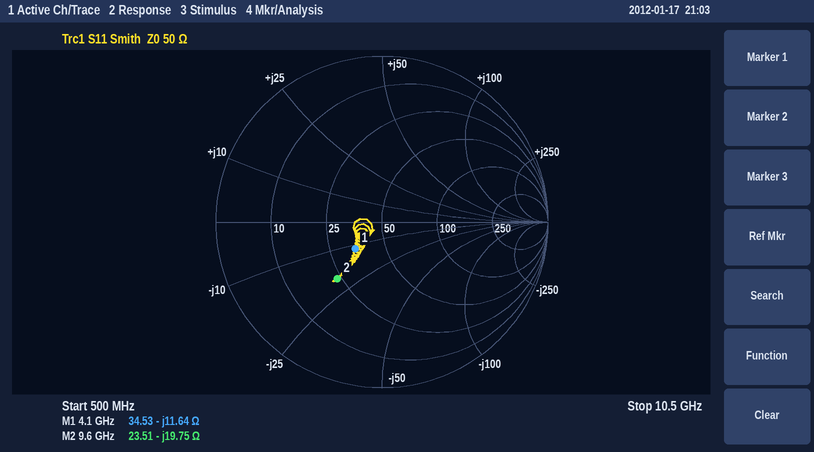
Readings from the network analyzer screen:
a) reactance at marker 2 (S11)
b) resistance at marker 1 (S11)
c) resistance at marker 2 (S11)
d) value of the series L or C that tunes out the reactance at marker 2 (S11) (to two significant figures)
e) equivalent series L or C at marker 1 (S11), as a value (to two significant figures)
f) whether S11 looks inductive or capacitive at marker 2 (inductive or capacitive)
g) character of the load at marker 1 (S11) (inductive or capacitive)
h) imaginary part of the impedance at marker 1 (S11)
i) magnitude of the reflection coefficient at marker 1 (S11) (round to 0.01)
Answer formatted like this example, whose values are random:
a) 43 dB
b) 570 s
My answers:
a) -19.75 Ω
b) 34.53 Ω
c) 23.51 Ω
d) 330 pH
e) 3.3 pF
f) capacitive
g) capacitive
h) -11.64 Ω
i) 0.23
